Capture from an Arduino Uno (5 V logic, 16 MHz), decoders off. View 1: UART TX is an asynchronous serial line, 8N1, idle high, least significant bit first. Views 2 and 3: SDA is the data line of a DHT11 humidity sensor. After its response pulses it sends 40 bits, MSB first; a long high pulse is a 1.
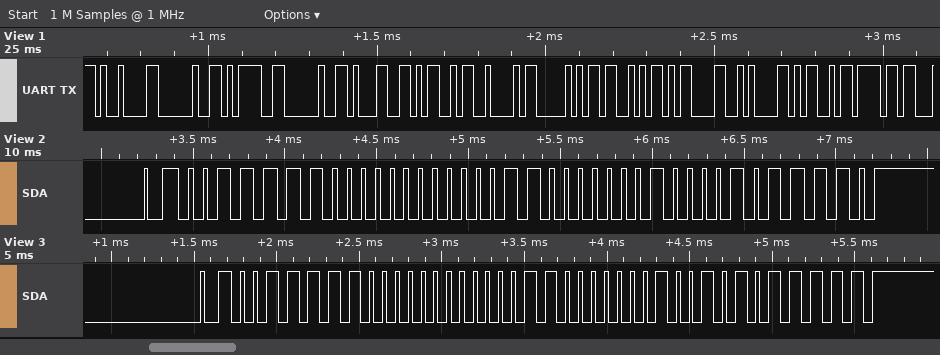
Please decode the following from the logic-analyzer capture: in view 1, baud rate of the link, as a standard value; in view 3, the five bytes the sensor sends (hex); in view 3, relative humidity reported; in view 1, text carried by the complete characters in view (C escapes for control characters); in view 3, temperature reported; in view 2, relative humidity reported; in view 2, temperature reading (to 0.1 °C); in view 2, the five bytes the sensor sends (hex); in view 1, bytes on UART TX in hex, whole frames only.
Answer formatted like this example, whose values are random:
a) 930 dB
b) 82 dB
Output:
a) 57600 baud
b) 3E 00 18 09 5F
c) 62 %
d) "\t = 1MBPS\r\nMo"
e) 24.9 °C
f) 62 %
g) 24.8 °C
h) 3E 00 18 08 5E
i) 0x09 0x20 0x3D 0x20 0x31 0x4D 0x42 0x50 0x53 0x0D 0x0A 0x4D 0x6F
